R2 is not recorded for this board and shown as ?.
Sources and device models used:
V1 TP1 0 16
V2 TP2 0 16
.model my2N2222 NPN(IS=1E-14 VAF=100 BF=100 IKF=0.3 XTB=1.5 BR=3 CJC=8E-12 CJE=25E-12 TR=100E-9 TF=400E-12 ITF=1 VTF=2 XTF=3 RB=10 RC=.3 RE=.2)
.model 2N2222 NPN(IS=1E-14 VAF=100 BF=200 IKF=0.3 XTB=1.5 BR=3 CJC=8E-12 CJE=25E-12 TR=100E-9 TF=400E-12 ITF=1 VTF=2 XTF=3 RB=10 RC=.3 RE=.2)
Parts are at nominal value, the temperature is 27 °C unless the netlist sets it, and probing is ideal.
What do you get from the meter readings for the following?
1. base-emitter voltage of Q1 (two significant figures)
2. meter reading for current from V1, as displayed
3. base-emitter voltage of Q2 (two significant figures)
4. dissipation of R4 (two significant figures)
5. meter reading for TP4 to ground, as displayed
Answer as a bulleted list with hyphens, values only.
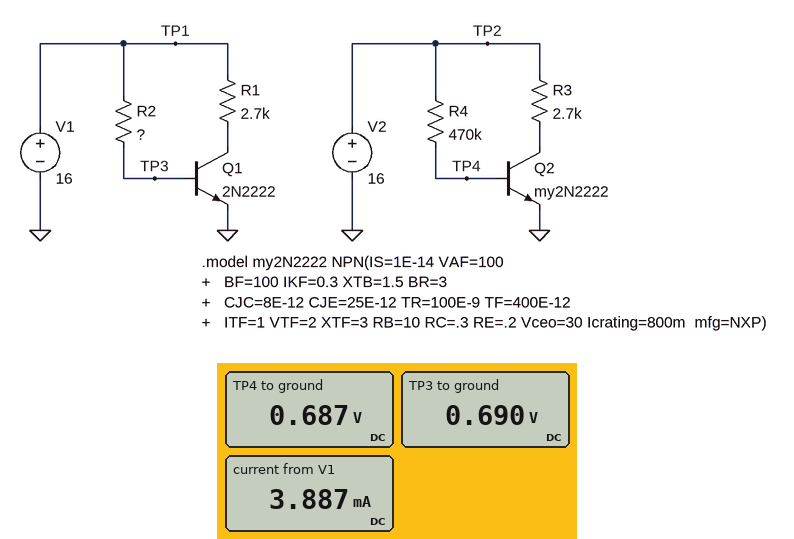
- 690 mV
- 3.887 mA
- 690 mV
- 500 µW
- 0.687 V
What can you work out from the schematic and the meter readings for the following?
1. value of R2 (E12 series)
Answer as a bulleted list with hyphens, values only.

- 820 kΩ
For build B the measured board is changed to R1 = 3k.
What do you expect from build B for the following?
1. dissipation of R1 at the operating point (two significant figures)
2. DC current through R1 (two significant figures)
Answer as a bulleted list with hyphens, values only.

- 44 mW
- 3.8 mA
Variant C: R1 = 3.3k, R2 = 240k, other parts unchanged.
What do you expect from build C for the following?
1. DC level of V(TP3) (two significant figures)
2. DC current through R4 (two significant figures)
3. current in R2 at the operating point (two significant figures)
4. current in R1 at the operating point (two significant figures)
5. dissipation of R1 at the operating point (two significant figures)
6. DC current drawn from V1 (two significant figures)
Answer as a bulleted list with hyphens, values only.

- 700 mV
- 33 µA
- 64 µA
- 4.8 mA
- 77 mW
- 4.9 mA
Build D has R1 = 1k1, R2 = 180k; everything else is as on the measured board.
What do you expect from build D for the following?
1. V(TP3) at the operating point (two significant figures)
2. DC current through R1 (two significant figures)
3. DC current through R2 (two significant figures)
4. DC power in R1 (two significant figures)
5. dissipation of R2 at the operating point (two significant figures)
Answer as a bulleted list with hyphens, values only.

- 730 mV
- 14 mA
- 85 µA
- 230 mW
- 1.3 mW
